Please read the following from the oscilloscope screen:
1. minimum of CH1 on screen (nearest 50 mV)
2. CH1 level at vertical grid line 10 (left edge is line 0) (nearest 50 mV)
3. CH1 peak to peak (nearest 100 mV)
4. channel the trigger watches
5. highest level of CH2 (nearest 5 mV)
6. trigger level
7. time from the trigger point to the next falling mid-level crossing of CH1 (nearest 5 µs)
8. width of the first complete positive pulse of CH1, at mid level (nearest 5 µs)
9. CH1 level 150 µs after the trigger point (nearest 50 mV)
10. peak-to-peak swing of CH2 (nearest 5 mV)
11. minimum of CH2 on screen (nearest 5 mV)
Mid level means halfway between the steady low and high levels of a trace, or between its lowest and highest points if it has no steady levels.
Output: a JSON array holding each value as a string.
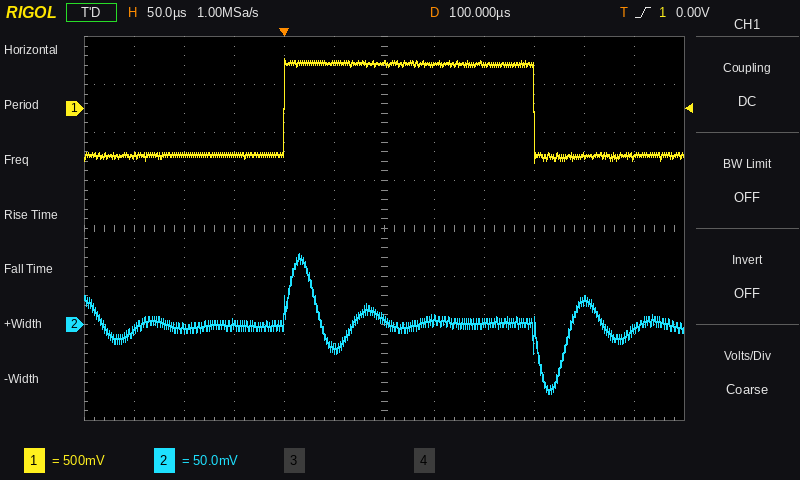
["-550 mV", "-500 mV", "1.10 V", "CH1", "75 mV", "0.00 V", "250 µs", "250 µs", "450 mV", "145 mV", "-70 mV"]
